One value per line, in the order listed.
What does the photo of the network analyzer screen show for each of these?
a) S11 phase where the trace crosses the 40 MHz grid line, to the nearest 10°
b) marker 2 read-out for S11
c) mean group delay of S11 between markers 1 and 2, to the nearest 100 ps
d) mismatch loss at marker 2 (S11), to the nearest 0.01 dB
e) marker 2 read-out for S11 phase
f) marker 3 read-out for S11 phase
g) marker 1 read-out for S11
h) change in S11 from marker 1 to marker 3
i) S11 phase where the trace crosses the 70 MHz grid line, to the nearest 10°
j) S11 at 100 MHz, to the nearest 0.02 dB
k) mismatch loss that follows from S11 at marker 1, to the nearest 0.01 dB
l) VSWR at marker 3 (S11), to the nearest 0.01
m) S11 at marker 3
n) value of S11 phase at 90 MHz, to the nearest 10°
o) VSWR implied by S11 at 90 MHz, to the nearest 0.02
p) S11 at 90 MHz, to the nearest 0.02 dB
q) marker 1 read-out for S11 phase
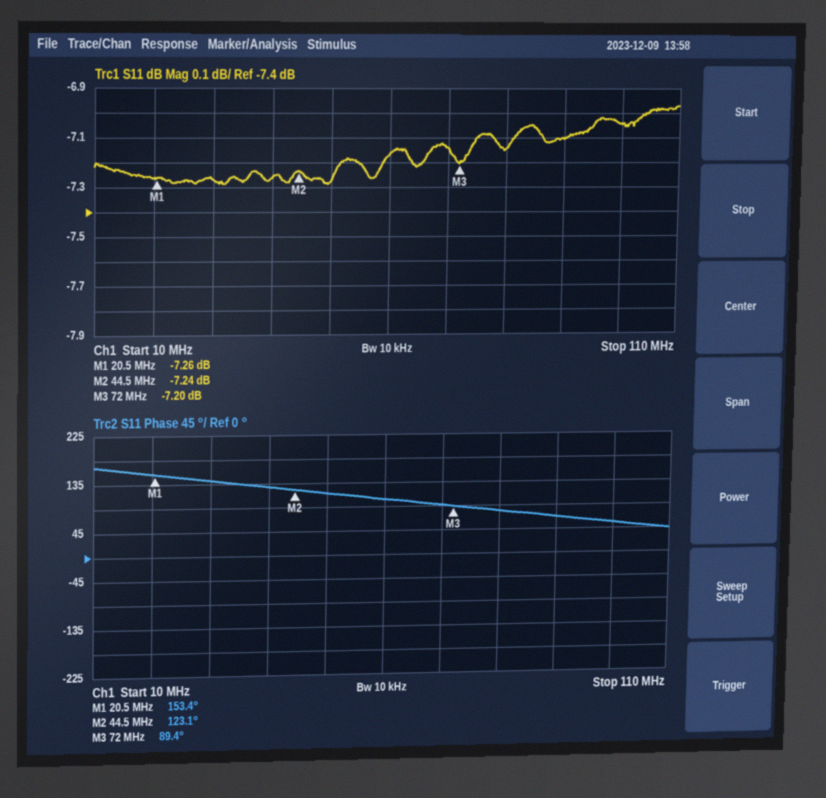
130°
-7.24 dB
3.5 ns
0.91 dB
123.1°
89.4°
-7.26 dB
0.06 dB
90°
-7.04 dB
0.90 dB
2.55
-7.20 dB
70°
2.58
-7.10 dB
153.4°
